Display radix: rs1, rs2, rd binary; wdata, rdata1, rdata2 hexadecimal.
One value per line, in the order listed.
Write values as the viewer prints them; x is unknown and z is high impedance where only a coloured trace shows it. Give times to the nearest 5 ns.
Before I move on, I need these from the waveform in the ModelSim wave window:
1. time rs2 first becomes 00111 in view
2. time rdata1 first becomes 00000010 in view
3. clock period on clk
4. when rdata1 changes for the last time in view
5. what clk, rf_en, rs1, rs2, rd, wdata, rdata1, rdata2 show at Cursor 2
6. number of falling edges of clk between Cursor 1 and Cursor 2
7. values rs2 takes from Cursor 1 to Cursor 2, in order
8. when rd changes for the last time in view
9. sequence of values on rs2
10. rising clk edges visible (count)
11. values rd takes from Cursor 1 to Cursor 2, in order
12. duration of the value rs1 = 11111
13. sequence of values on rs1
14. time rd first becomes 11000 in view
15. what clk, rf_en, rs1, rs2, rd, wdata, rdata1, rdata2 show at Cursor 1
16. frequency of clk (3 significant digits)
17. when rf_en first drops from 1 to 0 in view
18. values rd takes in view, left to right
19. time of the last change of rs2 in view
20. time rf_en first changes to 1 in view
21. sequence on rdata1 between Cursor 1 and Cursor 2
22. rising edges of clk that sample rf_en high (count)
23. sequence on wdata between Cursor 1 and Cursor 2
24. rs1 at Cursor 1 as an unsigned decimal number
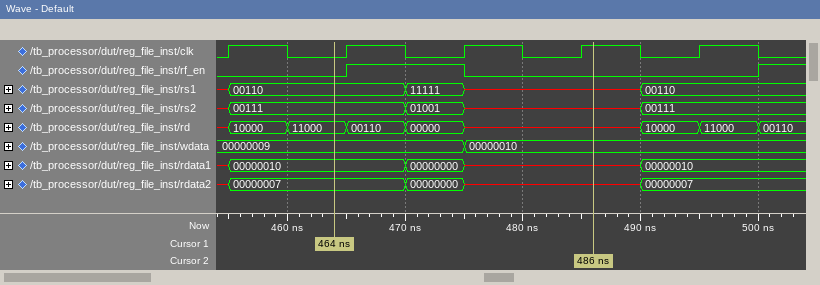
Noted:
455 ns
455 ns
10 ns
490 ns
clk=1, rf_en=0, rs1=x, rs2=x, rd=x, wdata=00000010, rdata1=x, rdata2=x
2
00111, 01001, x
500 ns
x, 00111, 01001, x, 00111
5
11000, 00110, 00000, x
5 ns
x, 00110, 11111, x, 00110
460 ns
clk=0, rf_en=0, rs1=00110, rs2=00111, rd=11000, wdata=00000009, rdata1=00000010, rdata2=00000007
100 MHz
475 ns
x, 10000, 11000, 00110, 00000, x, 10000, 11000, 00110
490 ns
465 ns
00000010, 00000000, x
1
00000009, 00000010
6
